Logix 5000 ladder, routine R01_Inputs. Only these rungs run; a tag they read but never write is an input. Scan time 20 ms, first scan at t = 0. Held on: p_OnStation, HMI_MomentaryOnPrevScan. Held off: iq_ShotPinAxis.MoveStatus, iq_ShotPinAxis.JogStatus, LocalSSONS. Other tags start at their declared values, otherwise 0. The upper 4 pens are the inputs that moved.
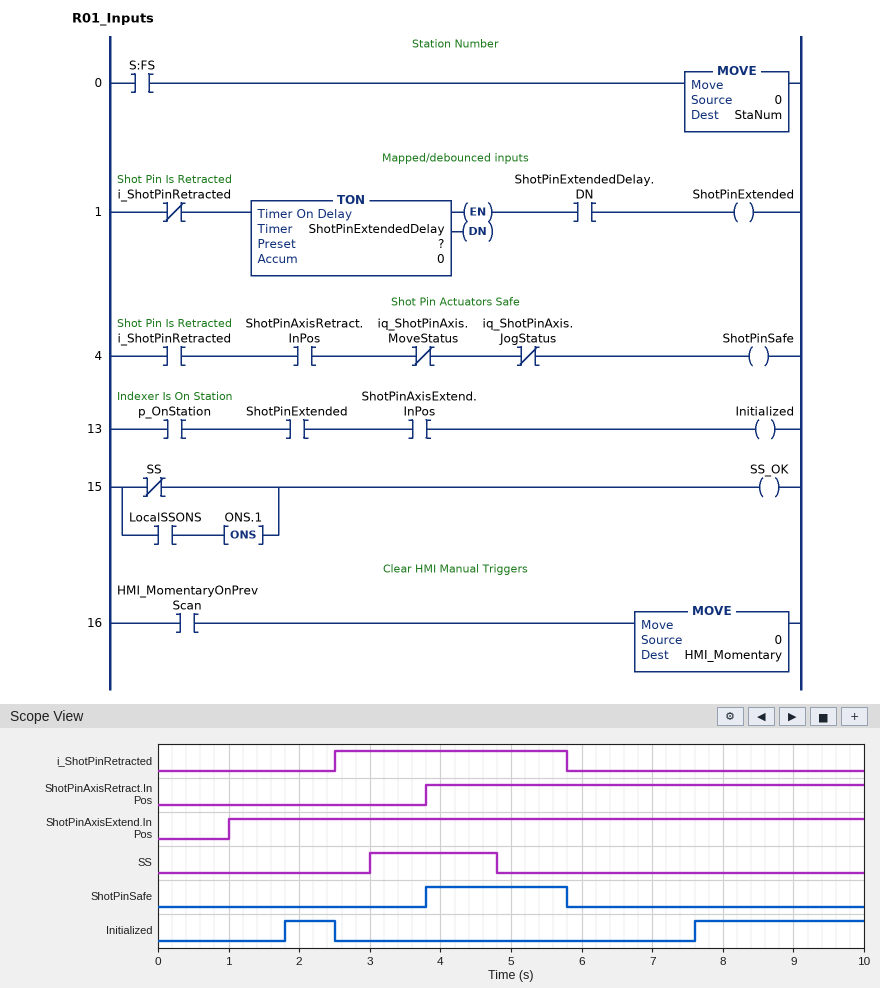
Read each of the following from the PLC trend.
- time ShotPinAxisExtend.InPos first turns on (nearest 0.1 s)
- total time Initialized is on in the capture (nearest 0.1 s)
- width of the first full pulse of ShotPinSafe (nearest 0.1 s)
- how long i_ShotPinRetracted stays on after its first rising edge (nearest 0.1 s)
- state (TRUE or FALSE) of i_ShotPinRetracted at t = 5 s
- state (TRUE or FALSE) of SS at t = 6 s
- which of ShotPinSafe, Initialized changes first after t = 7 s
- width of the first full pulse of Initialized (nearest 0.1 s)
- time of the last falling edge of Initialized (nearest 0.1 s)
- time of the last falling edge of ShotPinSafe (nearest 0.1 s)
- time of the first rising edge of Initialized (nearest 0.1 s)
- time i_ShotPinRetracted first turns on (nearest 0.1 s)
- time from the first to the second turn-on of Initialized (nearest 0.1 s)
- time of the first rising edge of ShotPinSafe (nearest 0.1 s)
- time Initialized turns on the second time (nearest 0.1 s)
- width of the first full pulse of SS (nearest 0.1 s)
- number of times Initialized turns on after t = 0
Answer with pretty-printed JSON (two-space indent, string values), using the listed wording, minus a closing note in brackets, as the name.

{
  "time ShotPinAxisExtend.InPos first turns on": "1.0 s",
  "total time Initialized is on in the capture": "3.1 s",
  "width of the first full pulse of ShotPinSafe": "2.0 s",
  "how long i_ShotPinRetracted stays on after its first rising edge": "3.3 s",
  "state (TRUE or FALSE) of i_ShotPinRetracted at t = 5 s": "TRUE",
  "state (TRUE or FALSE) of SS at t = 6 s": "FALSE",
  "which of ShotPinSafe, Initialized changes first after t = 7 s": "Initialized",
  "width of the first full pulse of Initialized": "0.7 s",
  "time of the last falling edge of Initialized": "2.5 s",
  "time of the last falling edge of ShotPinSafe": "5.8 s",
  "time of the first rising edge of Initialized": "1.8 s",
  "time i_ShotPinRetracted first turns on": "2.5 s",
  "time from the first to the second turn-on of Initialized": "5.8 s",
  "time of the first rising edge of ShotPinSafe": "3.8 s",
  "time Initialized turns on the second time": "7.6 s",
  "width of the first full pulse of SS": "1.8 s",
  "number of times Initialized turns on after t = 0": "2"
}
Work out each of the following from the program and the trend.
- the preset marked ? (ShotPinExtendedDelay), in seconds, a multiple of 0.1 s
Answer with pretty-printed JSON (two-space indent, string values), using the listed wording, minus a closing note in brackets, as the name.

{
  "the preset marked ? (ShotPinExtendedDelay), in seconds, a multiple of 0.1 s": "1.8 s"
}
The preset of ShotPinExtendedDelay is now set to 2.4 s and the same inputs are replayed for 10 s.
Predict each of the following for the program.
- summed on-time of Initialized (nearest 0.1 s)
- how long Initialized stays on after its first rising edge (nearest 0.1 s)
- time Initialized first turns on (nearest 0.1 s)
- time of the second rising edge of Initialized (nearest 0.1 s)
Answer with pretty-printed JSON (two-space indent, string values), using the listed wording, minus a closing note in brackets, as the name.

{
  "summed on-time of Initialized": "1.9 s",
  "how long Initialized stays on after its first rising edge": "0.1 s",
  "time Initialized first turns on": "2.4 s",
  "time of the second rising edge of Initialized": "8.2 s"
}
